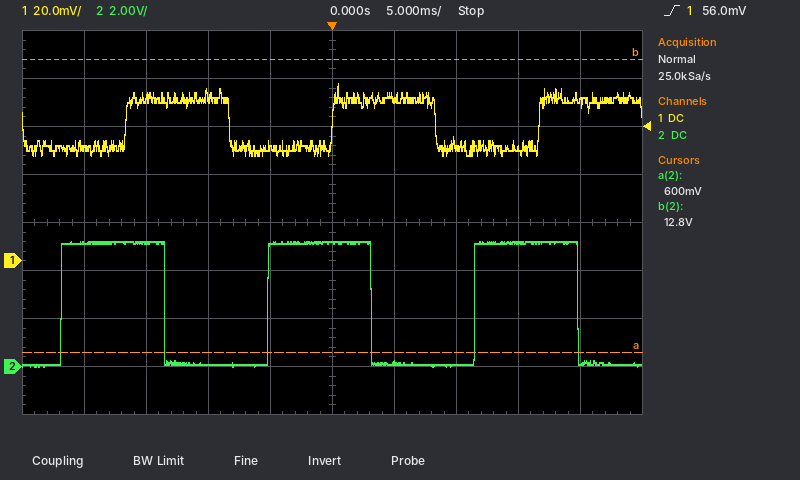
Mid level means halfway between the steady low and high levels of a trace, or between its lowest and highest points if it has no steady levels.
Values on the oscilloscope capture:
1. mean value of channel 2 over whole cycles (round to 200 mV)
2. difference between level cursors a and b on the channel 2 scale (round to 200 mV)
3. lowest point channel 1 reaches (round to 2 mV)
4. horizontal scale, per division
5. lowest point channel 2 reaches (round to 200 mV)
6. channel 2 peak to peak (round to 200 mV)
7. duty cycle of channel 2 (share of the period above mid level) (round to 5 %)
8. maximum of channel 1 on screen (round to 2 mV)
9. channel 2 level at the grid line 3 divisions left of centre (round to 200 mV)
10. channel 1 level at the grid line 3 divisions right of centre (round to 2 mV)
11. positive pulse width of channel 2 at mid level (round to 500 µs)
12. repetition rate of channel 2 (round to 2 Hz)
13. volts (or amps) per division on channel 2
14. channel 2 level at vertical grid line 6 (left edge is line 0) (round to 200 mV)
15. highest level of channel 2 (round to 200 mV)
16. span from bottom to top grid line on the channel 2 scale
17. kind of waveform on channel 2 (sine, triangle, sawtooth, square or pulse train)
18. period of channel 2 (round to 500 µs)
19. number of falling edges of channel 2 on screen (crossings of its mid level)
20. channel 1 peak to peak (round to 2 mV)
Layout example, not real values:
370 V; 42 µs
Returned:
2.6 V; 12.2 V; 44 mV; 5 ms; 0.0 V; 5.2 V; 50 %; 74 mV; 5.2 V; 46 mV; 8.5 ms; 60 Hz; 2 V; 200 mV; 5.2 V; 16 V; square; 16.5 ms; 3; 30 mV
